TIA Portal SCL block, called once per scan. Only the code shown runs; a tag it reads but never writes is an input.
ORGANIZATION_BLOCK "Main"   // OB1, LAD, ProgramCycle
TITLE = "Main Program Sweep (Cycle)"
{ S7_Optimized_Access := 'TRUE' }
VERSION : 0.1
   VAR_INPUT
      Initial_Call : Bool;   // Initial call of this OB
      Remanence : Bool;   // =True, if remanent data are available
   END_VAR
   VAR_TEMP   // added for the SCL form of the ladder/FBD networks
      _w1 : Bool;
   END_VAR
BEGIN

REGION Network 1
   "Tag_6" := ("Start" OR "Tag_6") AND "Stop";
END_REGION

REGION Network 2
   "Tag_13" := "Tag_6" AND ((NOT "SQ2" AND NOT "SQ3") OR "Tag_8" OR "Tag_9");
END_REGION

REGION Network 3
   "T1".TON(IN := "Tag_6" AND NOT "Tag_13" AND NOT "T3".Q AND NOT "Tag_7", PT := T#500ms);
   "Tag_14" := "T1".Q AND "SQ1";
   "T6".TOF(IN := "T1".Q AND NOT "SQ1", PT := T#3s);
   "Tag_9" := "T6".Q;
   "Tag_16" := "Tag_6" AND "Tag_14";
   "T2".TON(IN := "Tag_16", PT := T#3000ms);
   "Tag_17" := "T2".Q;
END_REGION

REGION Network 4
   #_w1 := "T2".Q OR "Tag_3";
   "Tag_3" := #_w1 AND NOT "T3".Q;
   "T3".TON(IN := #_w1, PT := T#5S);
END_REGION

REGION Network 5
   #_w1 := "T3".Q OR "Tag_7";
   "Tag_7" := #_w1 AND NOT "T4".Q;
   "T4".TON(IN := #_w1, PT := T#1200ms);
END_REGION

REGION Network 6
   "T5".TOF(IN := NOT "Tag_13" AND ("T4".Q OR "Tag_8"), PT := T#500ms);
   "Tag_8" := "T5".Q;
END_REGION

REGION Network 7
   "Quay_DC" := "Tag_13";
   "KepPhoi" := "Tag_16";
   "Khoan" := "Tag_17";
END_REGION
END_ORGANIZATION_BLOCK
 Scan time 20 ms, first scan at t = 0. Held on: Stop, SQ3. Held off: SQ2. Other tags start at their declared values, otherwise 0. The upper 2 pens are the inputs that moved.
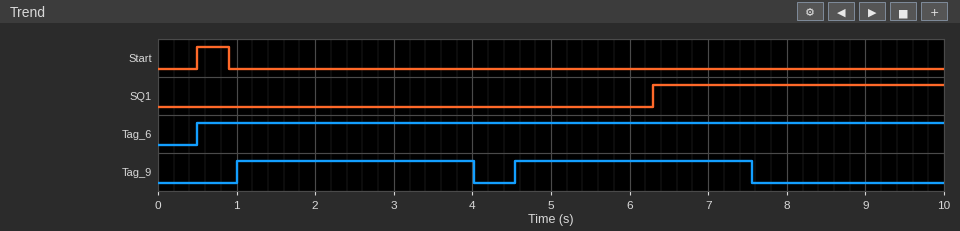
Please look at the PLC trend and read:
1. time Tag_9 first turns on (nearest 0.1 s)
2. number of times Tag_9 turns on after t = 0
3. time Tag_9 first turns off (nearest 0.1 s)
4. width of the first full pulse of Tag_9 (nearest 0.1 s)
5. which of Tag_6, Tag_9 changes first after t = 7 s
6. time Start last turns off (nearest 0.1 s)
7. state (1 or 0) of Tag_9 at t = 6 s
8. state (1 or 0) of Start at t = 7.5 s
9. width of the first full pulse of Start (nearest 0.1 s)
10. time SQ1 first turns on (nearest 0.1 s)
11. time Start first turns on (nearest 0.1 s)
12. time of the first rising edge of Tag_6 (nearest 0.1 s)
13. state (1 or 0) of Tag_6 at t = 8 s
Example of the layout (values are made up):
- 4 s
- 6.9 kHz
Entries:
- 1.0 s
- 2
- 4.0 s
- 3.0 s
- Tag_9
- 0.9 s
- 1
- 0
- 0.4 s
- 6.3 s
- 0.5 s
- 0.5 s
- 1
